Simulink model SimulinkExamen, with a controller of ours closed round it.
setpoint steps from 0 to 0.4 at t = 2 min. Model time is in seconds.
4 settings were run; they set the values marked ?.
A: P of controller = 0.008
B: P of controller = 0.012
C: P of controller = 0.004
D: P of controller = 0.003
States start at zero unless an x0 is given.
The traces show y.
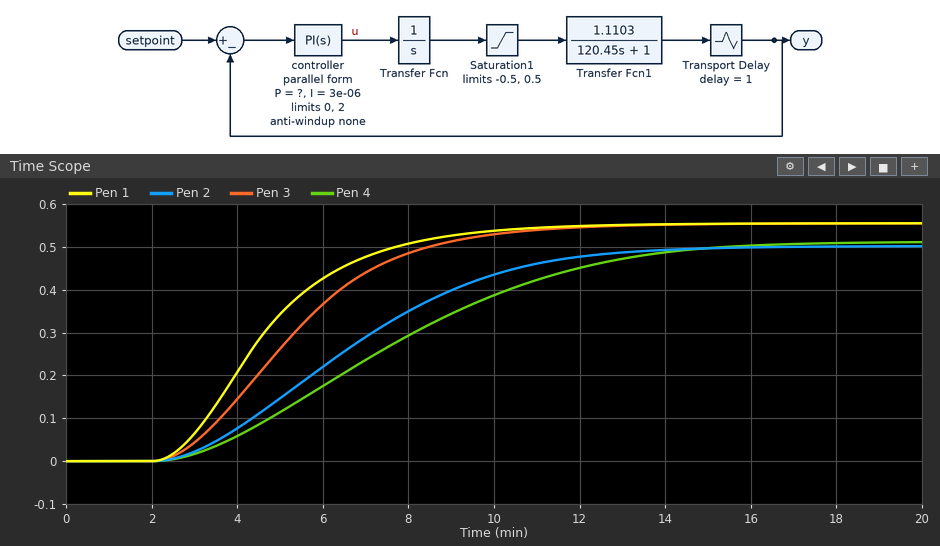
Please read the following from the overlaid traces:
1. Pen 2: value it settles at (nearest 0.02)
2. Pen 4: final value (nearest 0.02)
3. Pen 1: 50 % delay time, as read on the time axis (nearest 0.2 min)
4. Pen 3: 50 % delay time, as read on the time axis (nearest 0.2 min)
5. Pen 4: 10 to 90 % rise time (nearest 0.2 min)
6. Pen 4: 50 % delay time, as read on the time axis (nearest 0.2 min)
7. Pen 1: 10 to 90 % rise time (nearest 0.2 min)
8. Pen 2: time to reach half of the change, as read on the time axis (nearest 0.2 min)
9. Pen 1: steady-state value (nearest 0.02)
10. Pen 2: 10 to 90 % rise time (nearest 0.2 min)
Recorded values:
0.50
0.52
4.4 min
5.2 min
8.6 min
7.4 min
4.8 min
6.4 min
0.56
7.0 min
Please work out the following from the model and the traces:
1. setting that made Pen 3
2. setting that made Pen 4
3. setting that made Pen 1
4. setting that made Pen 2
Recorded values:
A
D
B
C
